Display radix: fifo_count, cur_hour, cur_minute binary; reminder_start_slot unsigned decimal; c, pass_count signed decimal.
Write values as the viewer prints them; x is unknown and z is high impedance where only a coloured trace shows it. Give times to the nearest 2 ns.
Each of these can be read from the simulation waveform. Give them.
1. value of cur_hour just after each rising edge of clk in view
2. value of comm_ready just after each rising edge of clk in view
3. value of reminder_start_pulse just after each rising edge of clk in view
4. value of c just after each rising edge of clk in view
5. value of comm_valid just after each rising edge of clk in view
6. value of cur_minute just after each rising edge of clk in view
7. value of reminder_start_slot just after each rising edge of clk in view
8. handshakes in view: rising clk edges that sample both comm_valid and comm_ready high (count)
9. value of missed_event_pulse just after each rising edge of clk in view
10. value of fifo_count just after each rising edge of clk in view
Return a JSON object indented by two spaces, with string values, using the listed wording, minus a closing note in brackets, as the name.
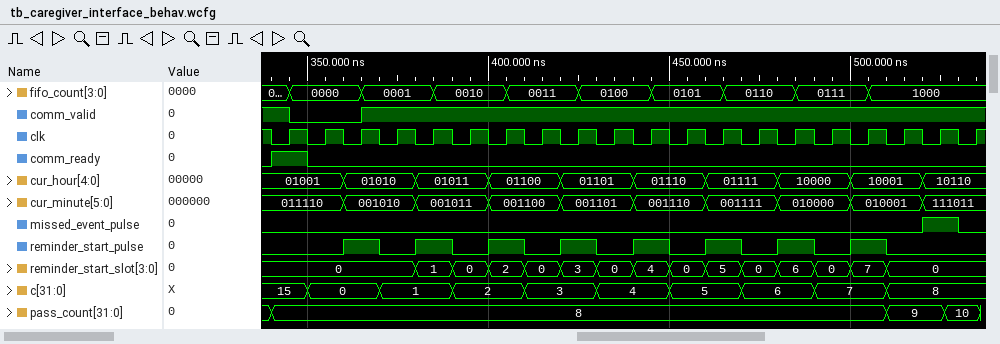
{
  "value of cur_hour just after each rising edge of clk in view": "01001, 01001, 01010, 01010, 01011, 01011, 01100, 01100, 01101, 01101, 01110, 01110, 01111, 01111, 10000, 10000, 10001, 10001, 10110, 10110",
  "value of comm_ready just after each rising edge of clk in view": "1 0 0 0 0 0 0 0 0 0 0 0 0 0 0 0 0 0 0 0",
  "value of reminder_start_pulse just after each rising edge of clk in view": "0 0 1 0 1 0 1 0 1 0 1 0 1 0 1 0 1 0 0 0",
  "value of c just after each rising edge of clk in view": "15, 0, 0, 1, 1, 2, 2, 3, 3, 4, 4, 5, 5, 6, 6, 7, 7, 8, 8, 8",
  "value of comm_valid just after each rising edge of clk in view": "0 0 1 1 1 1 1 1 1 1 1 1 1 1 1 1 1 1 1 1",
  "value of cur_minute just after each rising edge of clk in view": "011110, 011110, 001010, 001010, 001011, 001011, 001100, 001100, 001101, 001101, 001110, 001110, 001111, 001111, 010000, 010000, 010001, 010001, 111011, 111011",
  "value of reminder_start_slot just after each rising edge of clk in view": "0, 0, 0, 0, 1, 0, 2, 0, 3, 0, 4, 0, 5, 0, 6, 0, 7, 0, 0, 0",
  "handshakes in view: rising clk edges that sample both comm_valid and comm_ready high": "1",
  "value of missed_event_pulse just after each rising edge of clk in view": "0 0 0 0 0 0 0 0 0 0 0 0 0 0 0 0 0 0 1 0",
  "value of fifo_count just after each rising edge of clk in view": "0000, 0000, 0001, 0001, 0010, 0010, 0011, 0011, 0100, 0100, 0101, 0101, 0110, 0110, 0111, 0111, 1000, 1000, 1000, 1000"
}
